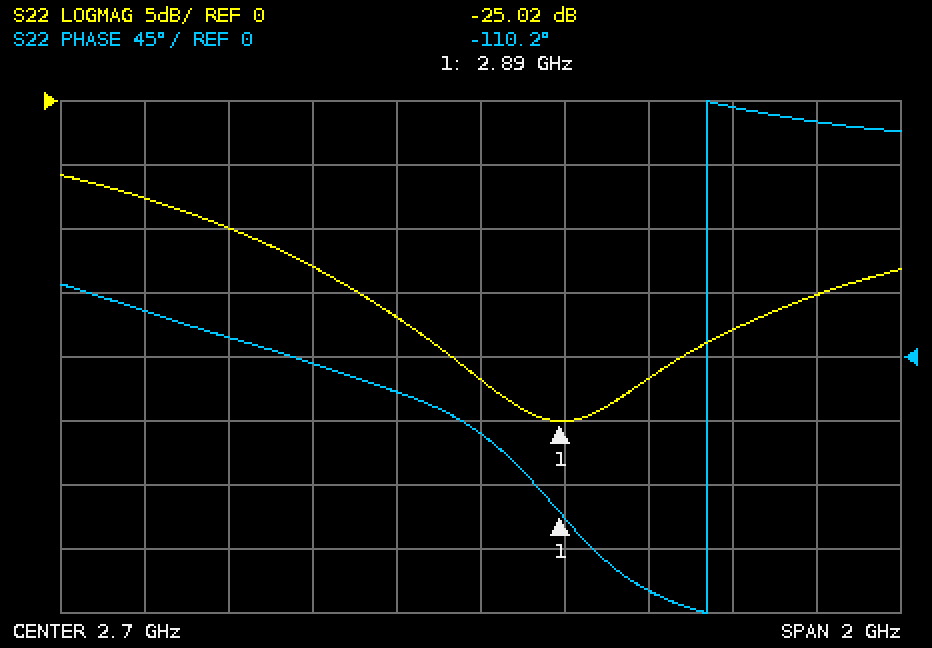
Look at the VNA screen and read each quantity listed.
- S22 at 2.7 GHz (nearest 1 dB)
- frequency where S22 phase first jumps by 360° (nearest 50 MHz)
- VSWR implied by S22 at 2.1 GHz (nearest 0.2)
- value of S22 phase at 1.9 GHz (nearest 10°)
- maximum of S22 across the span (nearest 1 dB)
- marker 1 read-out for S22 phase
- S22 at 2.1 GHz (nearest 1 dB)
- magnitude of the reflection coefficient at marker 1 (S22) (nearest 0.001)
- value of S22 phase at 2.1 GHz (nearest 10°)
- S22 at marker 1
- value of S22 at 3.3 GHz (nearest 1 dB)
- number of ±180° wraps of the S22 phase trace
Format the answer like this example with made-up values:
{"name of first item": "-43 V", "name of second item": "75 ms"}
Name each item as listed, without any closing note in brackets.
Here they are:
{"S22 at 2.7 GHz": "-22 dB", "frequency where S22 phase first jumps by 360°": "3.25 GHz", "VSWR implied by S22 at 2.1 GHz": "2.0", "value of S22 phase at 1.9 GHz": "30°", "maximum of S22 across the span": "-6 dB", "marker 1 read-out for S22 phase": "-110.2°", "S22 at 2.1 GHz": "-10 dB", "magnitude of the reflection coefficient at marker 1 (S22)": "0.056", "value of S22 phase at 2.1 GHz": "10°", "S22 at marker 1": "-25.02 dB", "value of S22 at 3.3 GHz": "-18 dB", "number of ±180° wraps of the S22 phase trace": "1"}
